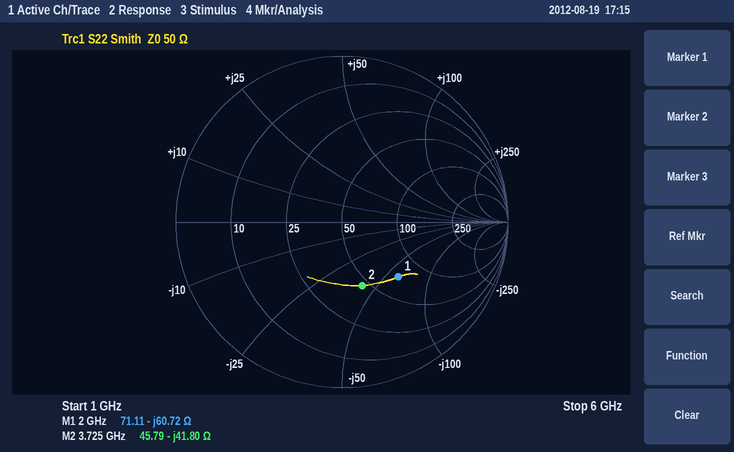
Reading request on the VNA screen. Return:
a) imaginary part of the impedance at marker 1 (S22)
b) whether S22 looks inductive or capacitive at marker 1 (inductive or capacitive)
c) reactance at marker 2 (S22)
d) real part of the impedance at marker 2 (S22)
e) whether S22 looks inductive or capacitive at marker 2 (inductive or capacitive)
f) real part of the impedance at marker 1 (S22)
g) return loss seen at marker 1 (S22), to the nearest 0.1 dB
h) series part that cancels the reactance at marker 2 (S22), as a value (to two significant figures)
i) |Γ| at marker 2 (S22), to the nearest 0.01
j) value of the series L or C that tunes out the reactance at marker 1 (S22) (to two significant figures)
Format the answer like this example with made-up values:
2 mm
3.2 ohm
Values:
-60.72 Ω
capacitive
-41.80 Ω
45.79 Ω
capacitive
71.11 Ω
6.5 dB
1.8 nH
0.40
4.8 nH
